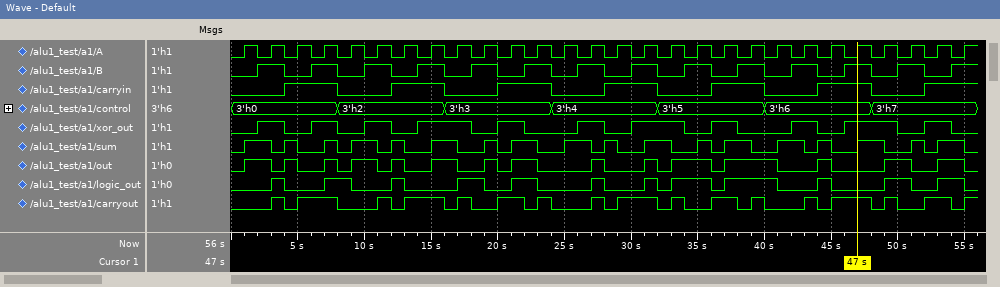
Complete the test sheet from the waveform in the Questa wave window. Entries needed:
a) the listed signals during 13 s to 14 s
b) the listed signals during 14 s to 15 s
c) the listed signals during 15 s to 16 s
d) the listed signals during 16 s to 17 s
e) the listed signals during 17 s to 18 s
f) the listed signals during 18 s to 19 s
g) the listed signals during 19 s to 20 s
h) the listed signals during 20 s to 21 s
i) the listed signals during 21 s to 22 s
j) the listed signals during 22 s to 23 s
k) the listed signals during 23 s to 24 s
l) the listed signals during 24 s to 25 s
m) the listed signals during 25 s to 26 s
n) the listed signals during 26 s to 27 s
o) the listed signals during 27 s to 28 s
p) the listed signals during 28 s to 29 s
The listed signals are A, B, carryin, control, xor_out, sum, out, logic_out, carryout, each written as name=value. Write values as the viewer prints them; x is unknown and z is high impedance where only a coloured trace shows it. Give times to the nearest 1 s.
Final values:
A=1, B=0, carryin=1, control=3'h2, xor_out=0, sum=0, out=0, logic_out=0, carryout=1
A=0, B=1, carryin=1, control=3'h2, xor_out=1, sum=0, out=0, logic_out=0, carryout=1
A=1, B=1, carryin=1, control=3'h2, xor_out=1, sum=1, out=1, logic_out=0, carryout=1
A=0, B=0, carryin=0, control=3'h3, xor_out=1, sum=1, out=1, logic_out=0, carryout=0
A=1, B=0, carryin=0, control=3'h3, xor_out=1, sum=0, out=0, logic_out=1, carryout=1
A=0, B=1, carryin=0, control=3'h3, xor_out=0, sum=0, out=0, logic_out=1, carryout=0
A=1, B=1, carryin=0, control=3'h3, xor_out=0, sum=1, out=1, logic_out=0, carryout=0
A=0, B=0, carryin=1, control=3'h3, xor_out=1, sum=0, out=0, logic_out=0, carryout=1
A=1, B=0, carryin=1, control=3'h3, xor_out=1, sum=1, out=1, logic_out=1, carryout=1
A=0, B=1, carryin=1, control=3'h3, xor_out=0, sum=1, out=1, logic_out=1, carryout=0
A=1, B=1, carryin=1, control=3'h3, xor_out=0, sum=0, out=0, logic_out=0, carryout=1
A=0, B=0, carryin=0, control=3'h4, xor_out=0, sum=0, out=0, logic_out=0, carryout=0
A=1, B=0, carryin=0, control=3'h4, xor_out=0, sum=1, out=0, logic_out=0, carryout=0
A=0, B=1, carryin=0, control=3'h4, xor_out=1, sum=1, out=0, logic_out=0, carryout=0
A=1, B=1, carryin=0, control=3'h4, xor_out=1, sum=0, out=1, logic_out=1, carryout=1
A=0, B=0, carryin=1, control=3'h4, xor_out=0, sum=1, out=0, logic_out=0, carryout=0
